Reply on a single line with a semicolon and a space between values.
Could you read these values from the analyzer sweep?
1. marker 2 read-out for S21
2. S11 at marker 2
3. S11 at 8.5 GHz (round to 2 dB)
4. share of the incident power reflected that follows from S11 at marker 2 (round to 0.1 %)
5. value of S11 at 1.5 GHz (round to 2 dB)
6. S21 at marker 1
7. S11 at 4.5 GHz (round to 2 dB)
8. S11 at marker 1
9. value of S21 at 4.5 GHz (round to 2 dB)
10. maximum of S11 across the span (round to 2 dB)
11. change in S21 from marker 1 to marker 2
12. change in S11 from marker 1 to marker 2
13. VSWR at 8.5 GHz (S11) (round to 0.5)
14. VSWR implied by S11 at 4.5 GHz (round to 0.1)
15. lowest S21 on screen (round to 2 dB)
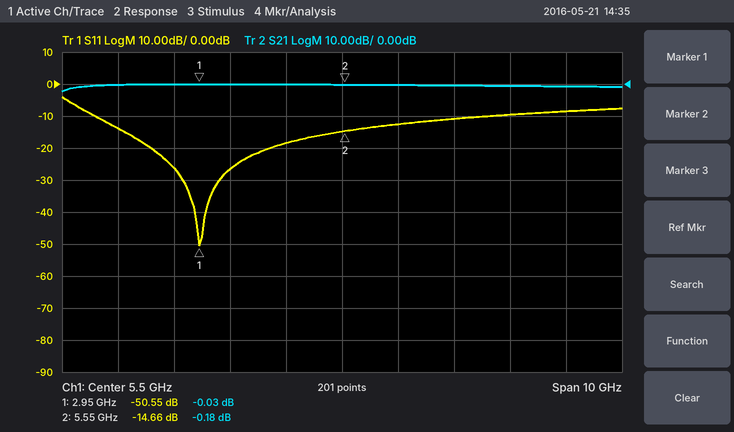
-0.18 dB; -14.66 dB; -10 dB; 3.4 %; -14 dB; -0.03 dB; -18 dB; -50.55 dB; 0 dB; -4 dB; -0.15 dB; 35.89 dB; 2.0; 1.3; -2 dB
